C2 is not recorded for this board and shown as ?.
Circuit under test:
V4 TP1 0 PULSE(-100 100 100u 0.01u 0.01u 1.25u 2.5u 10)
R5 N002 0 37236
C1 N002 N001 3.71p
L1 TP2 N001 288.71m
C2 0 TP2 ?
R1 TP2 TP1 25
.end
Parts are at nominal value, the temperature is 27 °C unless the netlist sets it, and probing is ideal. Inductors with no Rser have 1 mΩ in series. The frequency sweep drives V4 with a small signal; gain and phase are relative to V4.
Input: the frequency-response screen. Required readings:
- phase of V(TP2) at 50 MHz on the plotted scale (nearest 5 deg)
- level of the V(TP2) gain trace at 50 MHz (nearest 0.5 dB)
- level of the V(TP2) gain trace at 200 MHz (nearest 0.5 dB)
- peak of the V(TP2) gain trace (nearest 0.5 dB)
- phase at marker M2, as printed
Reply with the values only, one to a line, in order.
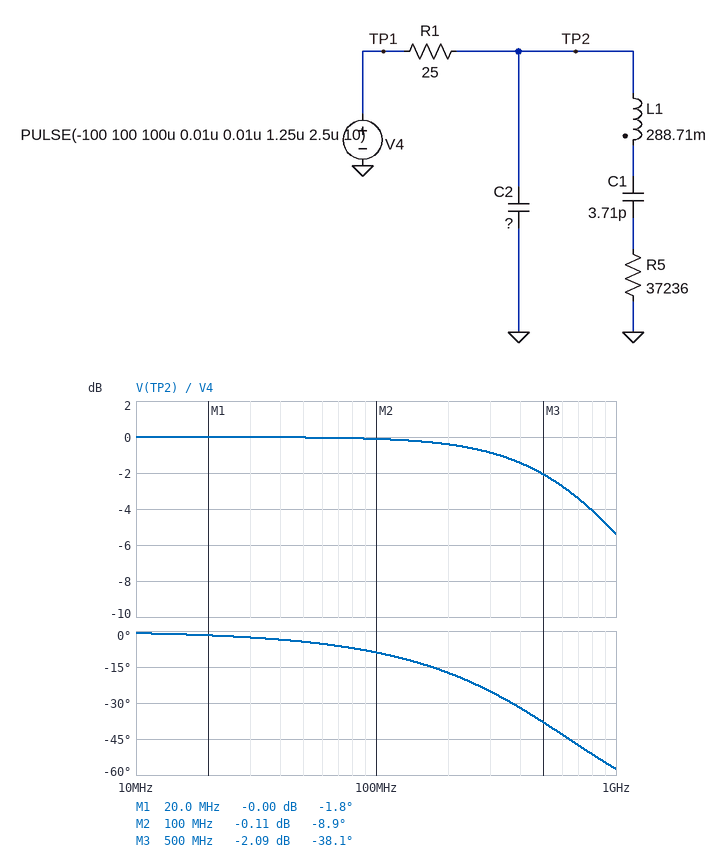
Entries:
-5 deg
0 dB
-0.5 dB
0 dB
-8.9 deg
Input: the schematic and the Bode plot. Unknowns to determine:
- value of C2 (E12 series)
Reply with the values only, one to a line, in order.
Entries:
10 pF
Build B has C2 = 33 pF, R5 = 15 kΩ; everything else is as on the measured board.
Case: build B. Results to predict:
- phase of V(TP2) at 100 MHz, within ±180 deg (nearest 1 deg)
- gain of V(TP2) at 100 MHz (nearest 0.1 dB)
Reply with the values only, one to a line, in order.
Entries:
-27 deg
-1.0 dB
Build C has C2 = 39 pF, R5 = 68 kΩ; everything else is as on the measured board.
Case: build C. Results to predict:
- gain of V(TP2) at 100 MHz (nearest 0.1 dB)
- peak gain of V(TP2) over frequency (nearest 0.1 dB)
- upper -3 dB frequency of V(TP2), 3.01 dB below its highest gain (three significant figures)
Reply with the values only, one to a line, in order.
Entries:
-1.4 dB
0 dB
163 MHz
